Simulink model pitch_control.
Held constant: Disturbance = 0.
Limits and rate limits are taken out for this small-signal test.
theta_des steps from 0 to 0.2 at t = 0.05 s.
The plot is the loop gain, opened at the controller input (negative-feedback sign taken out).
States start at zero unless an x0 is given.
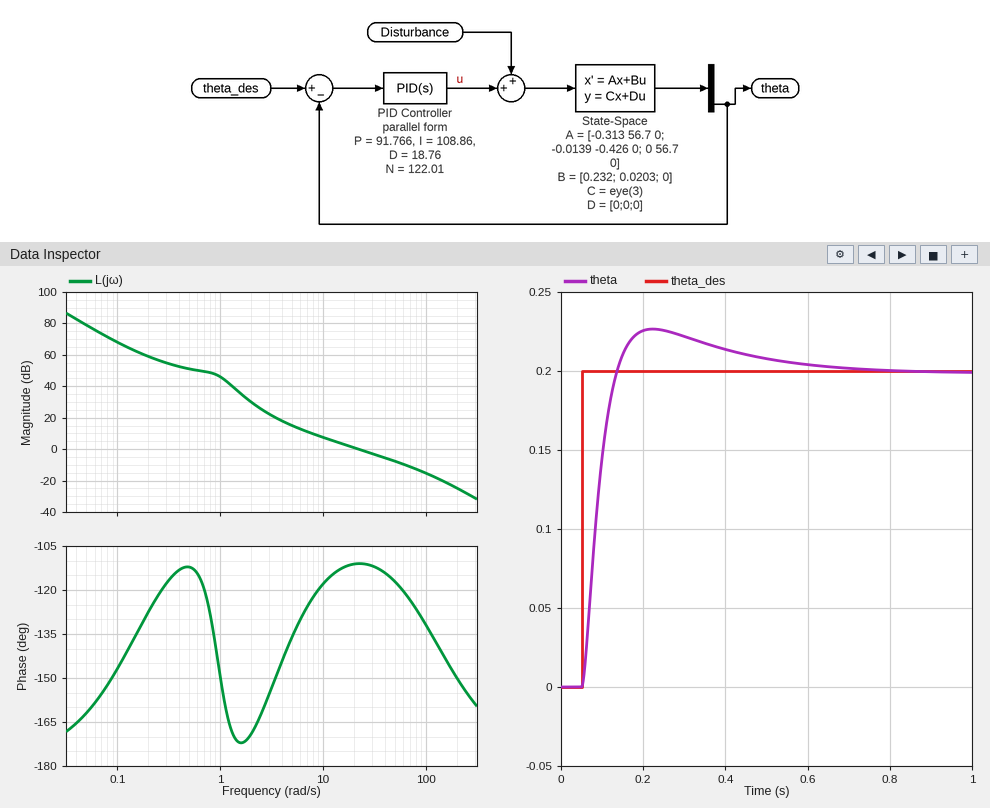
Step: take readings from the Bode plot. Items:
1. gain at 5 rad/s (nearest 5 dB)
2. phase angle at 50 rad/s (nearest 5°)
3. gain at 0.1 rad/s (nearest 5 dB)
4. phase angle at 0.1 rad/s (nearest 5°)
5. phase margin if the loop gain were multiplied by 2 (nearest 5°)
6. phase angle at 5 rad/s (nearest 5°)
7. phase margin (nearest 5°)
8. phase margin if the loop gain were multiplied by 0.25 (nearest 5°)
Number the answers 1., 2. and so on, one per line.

1. 15 dB
2. -115°
3. 70 dB
4. -145°
5. 65°
6. -135°
7. 70°
8. 50°
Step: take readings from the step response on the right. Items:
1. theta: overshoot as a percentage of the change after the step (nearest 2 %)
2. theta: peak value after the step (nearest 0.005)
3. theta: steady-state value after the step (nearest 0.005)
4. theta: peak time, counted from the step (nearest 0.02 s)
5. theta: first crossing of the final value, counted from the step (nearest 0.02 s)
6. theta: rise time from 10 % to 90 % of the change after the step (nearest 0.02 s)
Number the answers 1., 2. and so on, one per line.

1. 14 %
2. 0.225
3. 0.200
4. 0.18 s
5. 0.08 s
6. 0.06 s
